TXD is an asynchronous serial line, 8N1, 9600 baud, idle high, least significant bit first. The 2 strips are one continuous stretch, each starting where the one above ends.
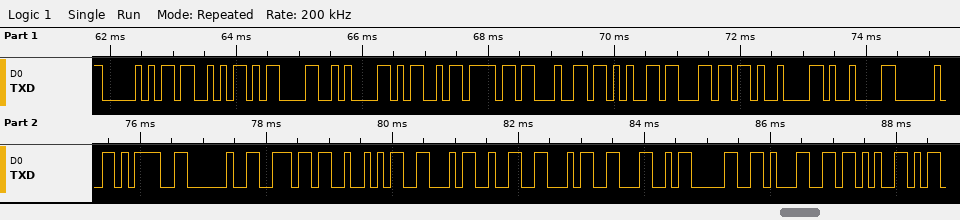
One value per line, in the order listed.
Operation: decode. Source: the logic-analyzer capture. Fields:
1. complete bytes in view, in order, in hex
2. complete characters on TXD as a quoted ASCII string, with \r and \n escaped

0x50 0x53 0x0D 0x0A 0x4D 0x6F 0x64 0x65 0x6C 0x09 0x09 0x20 0x3D 0x20 0x6E 0x52 0x46 0x32 0x34 0x4C 0x30 0x31 0x2B
"PS\r\nModel\t\t = nRF24L01+"
